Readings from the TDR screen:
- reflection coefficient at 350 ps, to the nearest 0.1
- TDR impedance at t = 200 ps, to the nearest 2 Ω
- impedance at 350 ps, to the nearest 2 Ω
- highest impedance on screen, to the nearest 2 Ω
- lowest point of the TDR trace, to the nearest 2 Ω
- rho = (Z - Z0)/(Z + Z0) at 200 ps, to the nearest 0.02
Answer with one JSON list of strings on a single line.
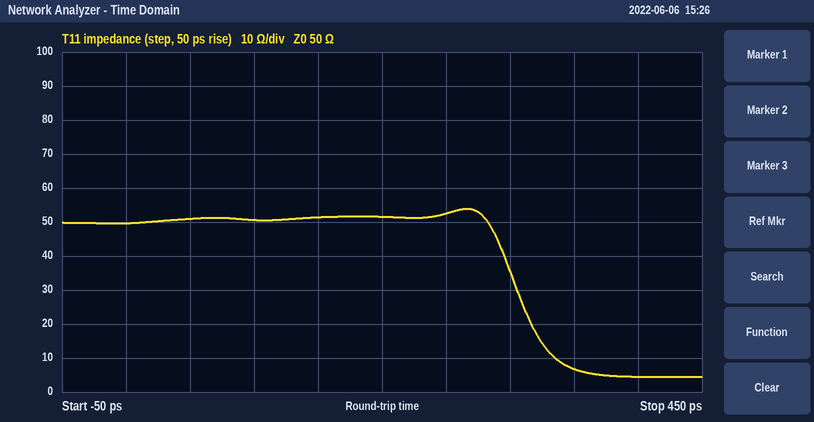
["-0.8", "52 Ω", "6 Ω", "54 Ω", "4 Ω", "+0.02"]
